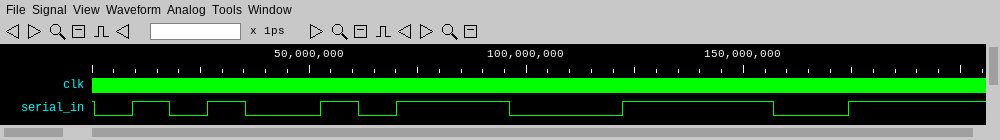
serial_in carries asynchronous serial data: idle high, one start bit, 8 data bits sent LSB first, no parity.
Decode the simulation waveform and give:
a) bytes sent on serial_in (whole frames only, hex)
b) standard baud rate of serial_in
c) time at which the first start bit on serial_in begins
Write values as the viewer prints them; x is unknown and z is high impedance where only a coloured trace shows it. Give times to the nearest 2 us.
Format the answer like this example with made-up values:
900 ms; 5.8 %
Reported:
A5, 3C; 115200 baud; 0 us
